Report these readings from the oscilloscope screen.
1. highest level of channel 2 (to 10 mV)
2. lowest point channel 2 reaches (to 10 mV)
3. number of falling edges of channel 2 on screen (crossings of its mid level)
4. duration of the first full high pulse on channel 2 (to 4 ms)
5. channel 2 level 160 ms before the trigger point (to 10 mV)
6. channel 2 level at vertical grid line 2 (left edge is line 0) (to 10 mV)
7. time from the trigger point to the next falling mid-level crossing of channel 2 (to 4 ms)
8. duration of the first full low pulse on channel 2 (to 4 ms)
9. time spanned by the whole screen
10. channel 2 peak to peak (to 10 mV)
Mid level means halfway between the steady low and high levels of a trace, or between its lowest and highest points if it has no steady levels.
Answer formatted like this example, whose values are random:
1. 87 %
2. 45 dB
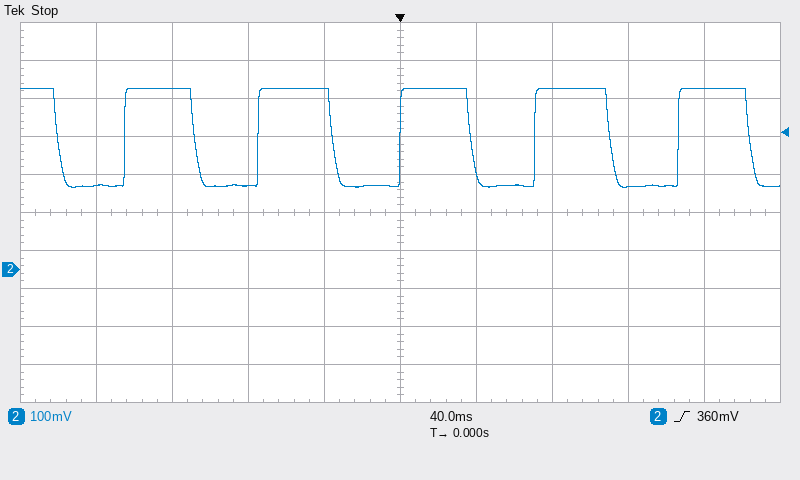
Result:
1. 480 mV
2. 220 mV
3. 6
4. 36 ms
5. 220 mV
6. 480 mV
7. 36 ms
8. 36 ms
9. 400 ms
10. 260 mV
